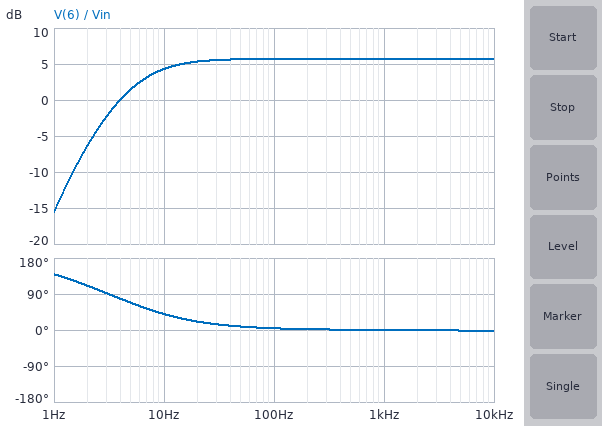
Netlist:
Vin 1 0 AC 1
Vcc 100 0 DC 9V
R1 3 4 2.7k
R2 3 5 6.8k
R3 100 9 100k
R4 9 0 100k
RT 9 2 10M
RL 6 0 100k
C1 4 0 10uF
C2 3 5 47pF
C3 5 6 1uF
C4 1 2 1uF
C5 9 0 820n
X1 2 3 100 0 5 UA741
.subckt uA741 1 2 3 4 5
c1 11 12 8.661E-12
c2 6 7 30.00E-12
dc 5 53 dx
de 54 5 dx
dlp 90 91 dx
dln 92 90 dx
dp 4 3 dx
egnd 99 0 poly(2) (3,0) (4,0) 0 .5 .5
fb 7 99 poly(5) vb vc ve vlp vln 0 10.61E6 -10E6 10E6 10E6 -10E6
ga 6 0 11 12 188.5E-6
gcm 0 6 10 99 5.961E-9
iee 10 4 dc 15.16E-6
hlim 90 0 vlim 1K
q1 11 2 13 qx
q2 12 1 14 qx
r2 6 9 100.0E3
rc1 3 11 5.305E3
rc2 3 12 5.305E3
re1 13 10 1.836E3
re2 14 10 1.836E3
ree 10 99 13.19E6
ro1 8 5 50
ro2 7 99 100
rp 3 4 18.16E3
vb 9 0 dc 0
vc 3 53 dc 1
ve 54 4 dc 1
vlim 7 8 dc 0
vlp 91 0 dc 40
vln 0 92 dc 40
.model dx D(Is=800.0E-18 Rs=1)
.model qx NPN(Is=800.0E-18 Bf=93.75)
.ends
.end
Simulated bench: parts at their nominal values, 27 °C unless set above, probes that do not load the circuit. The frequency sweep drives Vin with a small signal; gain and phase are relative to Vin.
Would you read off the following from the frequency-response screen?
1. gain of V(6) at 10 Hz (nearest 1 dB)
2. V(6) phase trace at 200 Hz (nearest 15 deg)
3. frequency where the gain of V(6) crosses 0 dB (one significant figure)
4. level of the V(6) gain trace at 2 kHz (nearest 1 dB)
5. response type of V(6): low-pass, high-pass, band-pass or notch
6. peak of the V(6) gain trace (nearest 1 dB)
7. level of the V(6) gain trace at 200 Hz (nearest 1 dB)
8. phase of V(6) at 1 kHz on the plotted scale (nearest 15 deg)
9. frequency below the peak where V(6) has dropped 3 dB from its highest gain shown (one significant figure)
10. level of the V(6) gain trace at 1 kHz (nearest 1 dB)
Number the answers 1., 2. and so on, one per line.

1. 4 dB
2. 0 deg
3. 4 Hz
4. 6 dB
5. high-pass
6. 6 dB
7. 6 dB
8. 0 deg
9. 6 Hz
10. 6 dB
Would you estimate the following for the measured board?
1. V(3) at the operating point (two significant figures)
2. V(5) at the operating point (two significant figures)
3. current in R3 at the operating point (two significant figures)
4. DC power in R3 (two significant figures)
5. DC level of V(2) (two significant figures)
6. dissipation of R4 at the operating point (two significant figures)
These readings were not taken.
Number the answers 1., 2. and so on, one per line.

1. 4.5 V
2. 4.5 V
3. 45 µA
4. 200 µW
5. 4.5 V
6. 200 µW
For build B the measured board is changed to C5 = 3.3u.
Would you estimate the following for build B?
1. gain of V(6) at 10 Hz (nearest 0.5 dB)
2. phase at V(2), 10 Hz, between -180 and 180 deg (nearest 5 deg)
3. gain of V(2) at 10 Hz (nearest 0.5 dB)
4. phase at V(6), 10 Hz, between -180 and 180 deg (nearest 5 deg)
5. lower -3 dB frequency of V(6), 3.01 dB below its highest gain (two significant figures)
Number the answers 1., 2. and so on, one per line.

1. -3.0 dB
2. 5 deg
3. -12.5 dB
4. 35 deg
5. 5.9 Hz
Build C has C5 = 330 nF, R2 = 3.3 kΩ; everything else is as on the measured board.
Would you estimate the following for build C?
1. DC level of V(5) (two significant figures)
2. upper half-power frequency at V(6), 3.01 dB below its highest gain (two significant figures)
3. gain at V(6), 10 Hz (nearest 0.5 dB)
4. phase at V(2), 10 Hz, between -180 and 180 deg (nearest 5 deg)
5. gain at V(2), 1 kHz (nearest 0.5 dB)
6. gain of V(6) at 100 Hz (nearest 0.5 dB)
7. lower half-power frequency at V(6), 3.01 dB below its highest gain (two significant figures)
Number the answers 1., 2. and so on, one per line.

1. 4.5 V
2. 420 kHz
3. 3.0 dB
4. 15 deg
5. -2.5 dB
6. 4.5 dB
7. 6.1 Hz
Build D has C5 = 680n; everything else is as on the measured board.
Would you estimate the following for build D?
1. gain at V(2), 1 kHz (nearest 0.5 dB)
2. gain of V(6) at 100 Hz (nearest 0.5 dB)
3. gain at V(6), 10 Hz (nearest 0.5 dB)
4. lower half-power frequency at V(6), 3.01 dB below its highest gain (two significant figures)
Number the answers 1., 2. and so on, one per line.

1. -4.5 dB
2. 6.5 dB
3. 5.0 dB
4. 6.4 Hz
